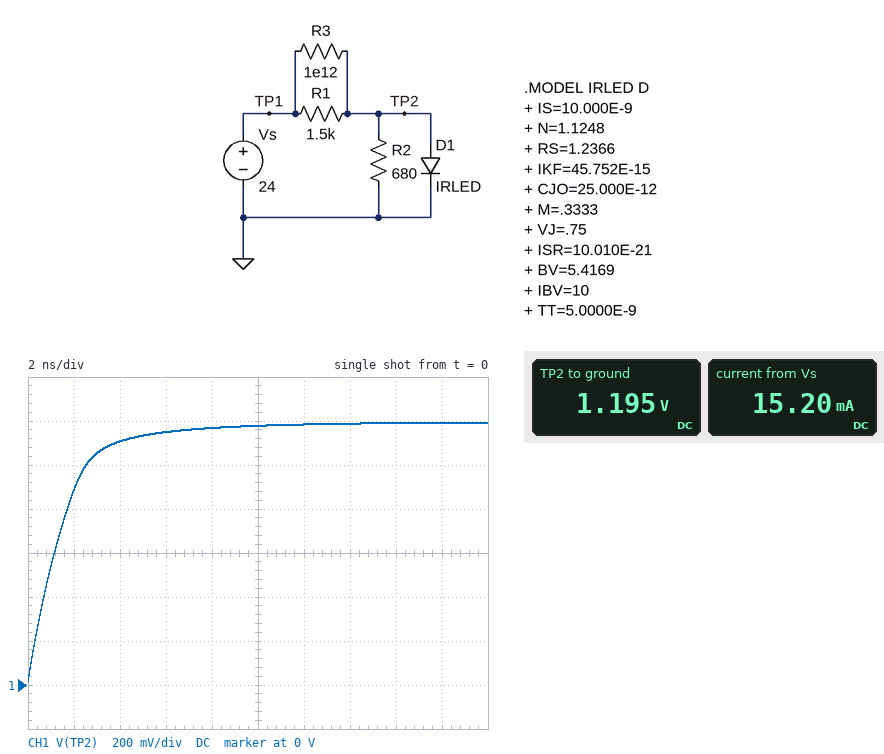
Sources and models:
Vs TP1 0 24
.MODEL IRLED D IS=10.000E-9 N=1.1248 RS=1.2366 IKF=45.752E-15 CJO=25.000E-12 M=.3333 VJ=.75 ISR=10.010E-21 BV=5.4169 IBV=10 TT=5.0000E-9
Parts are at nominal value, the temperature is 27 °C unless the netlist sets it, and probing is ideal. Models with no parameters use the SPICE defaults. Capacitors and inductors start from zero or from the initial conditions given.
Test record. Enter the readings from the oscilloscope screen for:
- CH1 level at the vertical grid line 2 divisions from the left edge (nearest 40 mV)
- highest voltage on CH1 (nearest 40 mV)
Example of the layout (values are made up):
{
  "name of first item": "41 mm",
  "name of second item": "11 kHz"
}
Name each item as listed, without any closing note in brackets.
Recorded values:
{
  "CH1 level at the vertical grid line 2 divisions from the left edge": "1.12 V",
  "highest voltage on CH1": "1.20 V"
}
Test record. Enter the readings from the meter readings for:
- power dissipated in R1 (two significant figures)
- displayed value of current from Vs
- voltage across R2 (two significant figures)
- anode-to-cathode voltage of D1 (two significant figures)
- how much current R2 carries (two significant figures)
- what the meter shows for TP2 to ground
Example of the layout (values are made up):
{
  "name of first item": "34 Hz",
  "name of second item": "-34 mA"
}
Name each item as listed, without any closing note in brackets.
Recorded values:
{
  "power dissipated in R1": "350 mW",
  "displayed value of current from Vs": "15.20 mA",
  "voltage across R2": "1.2 V",
  "anode-to-cathode voltage of D1": "1.2 V",
  "how much current R2 carries": "1.8 mA",
  "what the meter shows for TP2 to ground": "1.195 V"
}
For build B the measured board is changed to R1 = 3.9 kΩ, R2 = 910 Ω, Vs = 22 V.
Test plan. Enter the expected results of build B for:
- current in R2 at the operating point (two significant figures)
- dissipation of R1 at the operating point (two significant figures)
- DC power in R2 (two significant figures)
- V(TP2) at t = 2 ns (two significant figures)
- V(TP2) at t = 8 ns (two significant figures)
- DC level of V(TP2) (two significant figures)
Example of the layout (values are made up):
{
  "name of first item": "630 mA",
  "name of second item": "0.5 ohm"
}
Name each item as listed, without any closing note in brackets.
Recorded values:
{
  "current in R2 at the operating point": "1.2 mA",
  "dissipation of R1 at the operating point": "110 mW",
  "DC power in R2": "1.4 mW",
  "V(TP2) at t = 2 ns": "390 mV",
  "V(TP2) at t = 8 ns": "1.0 V",
  "DC level of V(TP2)": "1.1 V"
}
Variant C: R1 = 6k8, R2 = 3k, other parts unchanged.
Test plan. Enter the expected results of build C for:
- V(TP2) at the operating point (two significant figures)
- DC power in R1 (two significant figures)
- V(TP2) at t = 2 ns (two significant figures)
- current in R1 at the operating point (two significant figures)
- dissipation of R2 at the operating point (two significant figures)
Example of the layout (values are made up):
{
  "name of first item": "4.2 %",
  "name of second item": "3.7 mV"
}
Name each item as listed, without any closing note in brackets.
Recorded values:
{
  "V(TP2) at the operating point": "1.1 V",
  "DC power in R1": "77 mW",
  "V(TP2) at t = 2 ns": "260 mV",
  "current in R1 at the operating point": "3.4 mA",
  "dissipation of R2 at the operating point": "400 µW"
}
